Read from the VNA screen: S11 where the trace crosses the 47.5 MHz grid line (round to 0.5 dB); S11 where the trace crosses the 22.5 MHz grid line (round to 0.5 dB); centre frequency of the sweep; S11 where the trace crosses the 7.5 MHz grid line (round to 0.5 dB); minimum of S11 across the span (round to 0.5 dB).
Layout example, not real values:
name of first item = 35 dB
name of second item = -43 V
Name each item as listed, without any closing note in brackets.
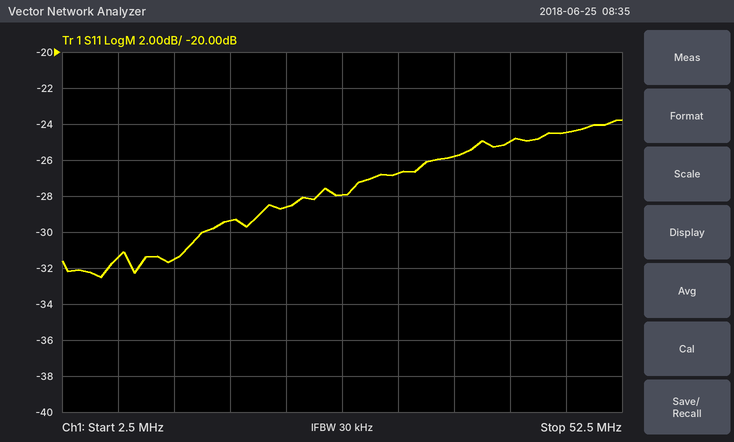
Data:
S11 where the trace crosses the 47.5 MHz grid line = -24.5 dB
S11 where the trace crosses the 22.5 MHz grid line = -28.5 dB
centre frequency of the sweep = 27.5 MHz
S11 where the trace crosses the 7.5 MHz grid line = -31.5 dB
minimum of S11 across the span = -32.5 dB
